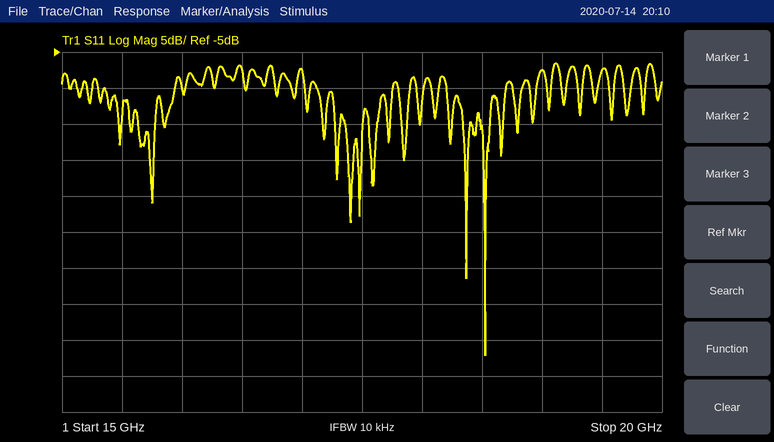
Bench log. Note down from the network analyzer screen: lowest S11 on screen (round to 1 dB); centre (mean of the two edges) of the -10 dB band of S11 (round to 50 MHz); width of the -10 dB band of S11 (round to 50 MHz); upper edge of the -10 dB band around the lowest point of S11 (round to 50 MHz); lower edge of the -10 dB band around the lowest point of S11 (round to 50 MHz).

-47 dB
18.45 GHz
500 MHz
18.70 GHz
18.20 GHz
